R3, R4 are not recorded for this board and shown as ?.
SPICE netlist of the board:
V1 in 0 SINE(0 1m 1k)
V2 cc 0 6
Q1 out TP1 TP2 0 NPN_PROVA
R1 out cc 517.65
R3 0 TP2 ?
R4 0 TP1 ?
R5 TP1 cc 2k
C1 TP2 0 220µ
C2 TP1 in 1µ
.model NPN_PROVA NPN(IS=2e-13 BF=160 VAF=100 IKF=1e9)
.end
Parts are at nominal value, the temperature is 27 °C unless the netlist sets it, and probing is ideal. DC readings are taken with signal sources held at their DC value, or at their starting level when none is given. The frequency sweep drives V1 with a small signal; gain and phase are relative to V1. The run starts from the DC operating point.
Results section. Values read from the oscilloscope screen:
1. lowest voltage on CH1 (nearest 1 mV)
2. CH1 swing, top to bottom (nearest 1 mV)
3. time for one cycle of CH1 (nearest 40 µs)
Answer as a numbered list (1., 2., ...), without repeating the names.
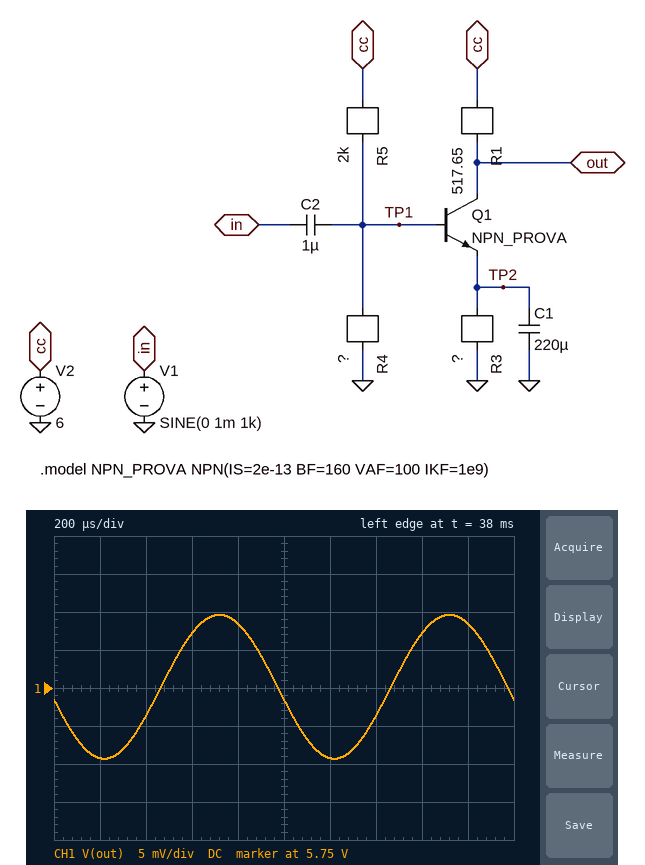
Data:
1. 5.741 V
2. 19 mV
3. 1.00 ms
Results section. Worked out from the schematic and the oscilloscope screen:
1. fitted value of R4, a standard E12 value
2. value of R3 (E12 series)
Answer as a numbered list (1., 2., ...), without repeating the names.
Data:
1. 1.8 kΩ
2. 4.7 kΩ
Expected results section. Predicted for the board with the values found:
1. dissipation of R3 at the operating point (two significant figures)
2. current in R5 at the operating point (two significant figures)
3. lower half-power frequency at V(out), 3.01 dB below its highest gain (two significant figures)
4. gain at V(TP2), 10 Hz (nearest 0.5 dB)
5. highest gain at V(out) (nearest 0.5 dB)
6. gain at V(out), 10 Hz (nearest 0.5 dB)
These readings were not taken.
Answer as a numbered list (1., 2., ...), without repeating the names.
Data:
1. 1.1 mW
2. 1.6 mA
3. 190 Hz
4. -27.0 dB
5. 19.5 dB
6. -10.0 dB
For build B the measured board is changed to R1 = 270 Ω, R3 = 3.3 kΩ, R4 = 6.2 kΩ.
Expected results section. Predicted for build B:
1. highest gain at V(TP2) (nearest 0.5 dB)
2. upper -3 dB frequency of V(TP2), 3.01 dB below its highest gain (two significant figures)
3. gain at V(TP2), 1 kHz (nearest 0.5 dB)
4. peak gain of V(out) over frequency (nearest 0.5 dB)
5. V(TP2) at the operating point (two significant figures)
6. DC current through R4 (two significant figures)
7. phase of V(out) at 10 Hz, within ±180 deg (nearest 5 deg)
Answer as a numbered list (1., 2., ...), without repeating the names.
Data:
1. -15.0 dB
2. 200 Hz
3. -29.5 dB
4. 22.0 dB
5. 3.9 V
6. 730 µA
7. -30 deg
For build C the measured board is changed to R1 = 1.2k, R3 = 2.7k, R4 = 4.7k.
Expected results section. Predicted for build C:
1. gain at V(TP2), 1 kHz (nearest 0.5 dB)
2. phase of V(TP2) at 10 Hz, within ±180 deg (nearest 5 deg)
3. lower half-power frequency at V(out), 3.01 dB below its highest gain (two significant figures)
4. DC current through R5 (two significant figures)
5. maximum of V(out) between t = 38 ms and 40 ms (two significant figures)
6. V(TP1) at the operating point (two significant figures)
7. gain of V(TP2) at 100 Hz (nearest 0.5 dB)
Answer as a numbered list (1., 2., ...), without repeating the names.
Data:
1. -29.0 dB
2. 65 deg
3. 180 Hz
4. 900 µA
5. 4.5 V
6. 4.2 V
7. -15.0 dB
